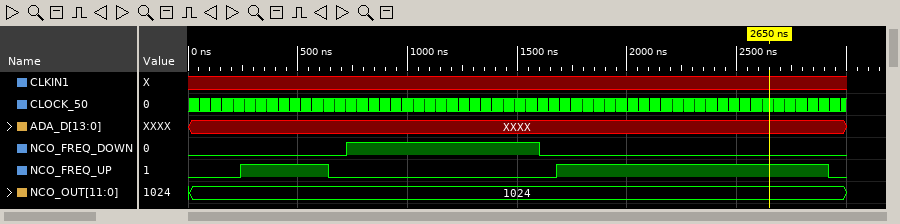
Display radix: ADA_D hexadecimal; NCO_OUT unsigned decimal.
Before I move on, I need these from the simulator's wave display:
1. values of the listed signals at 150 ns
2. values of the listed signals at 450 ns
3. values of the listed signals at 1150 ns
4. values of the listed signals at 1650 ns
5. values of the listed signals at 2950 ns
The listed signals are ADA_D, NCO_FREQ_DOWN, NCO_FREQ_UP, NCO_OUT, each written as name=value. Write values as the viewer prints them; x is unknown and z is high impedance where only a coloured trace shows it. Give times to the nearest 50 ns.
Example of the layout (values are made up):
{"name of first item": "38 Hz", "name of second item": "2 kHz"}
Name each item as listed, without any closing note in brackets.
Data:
{"values of the listed signals at 150 ns": "ADA_D=XXXX, NCO_FREQ_DOWN=0, NCO_FREQ_UP=0, NCO_OUT=1024", "values of the listed signals at 450 ns": "ADA_D=XXXX, NCO_FREQ_DOWN=0, NCO_FREQ_UP=1, NCO_OUT=1024", "values of the listed signals at 1150 ns": "ADA_D=XXXX, NCO_FREQ_DOWN=1, NCO_FREQ_UP=0, NCO_OUT=1024", "values of the listed signals at 1650 ns": "ADA_D=XXXX, NCO_FREQ_DOWN=0, NCO_FREQ_UP=0, NCO_OUT=1024", "values of the listed signals at 2950 ns": "ADA_D=XXXX, NCO_FREQ_DOWN=0, NCO_FREQ_UP=0, NCO_OUT=1024"}
